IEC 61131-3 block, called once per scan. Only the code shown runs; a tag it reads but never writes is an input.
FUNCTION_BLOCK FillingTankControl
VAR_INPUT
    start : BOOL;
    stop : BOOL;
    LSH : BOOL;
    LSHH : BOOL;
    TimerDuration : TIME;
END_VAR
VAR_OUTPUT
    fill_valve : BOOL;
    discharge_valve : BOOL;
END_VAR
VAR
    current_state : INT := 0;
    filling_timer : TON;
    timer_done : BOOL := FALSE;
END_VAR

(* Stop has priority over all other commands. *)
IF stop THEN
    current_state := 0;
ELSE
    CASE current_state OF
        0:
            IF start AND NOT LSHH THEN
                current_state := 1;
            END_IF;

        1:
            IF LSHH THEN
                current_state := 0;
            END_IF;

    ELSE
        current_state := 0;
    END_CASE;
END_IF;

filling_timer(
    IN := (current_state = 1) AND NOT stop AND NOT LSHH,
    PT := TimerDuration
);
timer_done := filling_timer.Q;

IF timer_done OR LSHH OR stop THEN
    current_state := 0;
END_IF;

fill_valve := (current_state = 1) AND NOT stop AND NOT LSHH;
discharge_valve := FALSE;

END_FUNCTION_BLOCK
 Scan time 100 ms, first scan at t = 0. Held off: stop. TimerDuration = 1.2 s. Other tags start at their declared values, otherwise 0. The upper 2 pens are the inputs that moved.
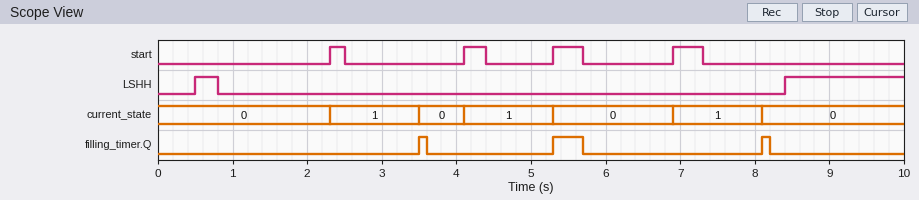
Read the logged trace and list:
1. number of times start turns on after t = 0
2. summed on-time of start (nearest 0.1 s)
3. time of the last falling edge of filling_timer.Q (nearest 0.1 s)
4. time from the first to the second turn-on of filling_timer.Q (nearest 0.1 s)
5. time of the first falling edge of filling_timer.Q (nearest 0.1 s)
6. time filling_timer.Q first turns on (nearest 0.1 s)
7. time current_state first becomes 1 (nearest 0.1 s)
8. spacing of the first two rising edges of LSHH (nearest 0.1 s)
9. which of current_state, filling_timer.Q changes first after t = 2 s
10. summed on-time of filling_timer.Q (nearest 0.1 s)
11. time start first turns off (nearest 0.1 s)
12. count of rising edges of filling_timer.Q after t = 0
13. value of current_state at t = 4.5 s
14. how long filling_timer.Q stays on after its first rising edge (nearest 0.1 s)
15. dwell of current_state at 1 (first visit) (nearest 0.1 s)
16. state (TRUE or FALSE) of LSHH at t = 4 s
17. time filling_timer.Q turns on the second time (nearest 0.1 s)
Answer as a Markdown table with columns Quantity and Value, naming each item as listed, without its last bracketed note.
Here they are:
| Quantity | Value |
|---|---|
| number of times start turns on after t = 0 | 4 |
| summed on-time of start | 1.3 s |
| time of the last falling edge of filling_timer.Q | 8.2 s |
| time from the first to the second turn-on of filling_timer.Q | 1.8 s |
| time of the first falling edge of filling_timer.Q | 3.6 s |
| time filling_timer.Q first turns on | 3.5 s |
| time current_state first becomes 1 | 2.3 s |
| spacing of the first two rising edges of LSHH | 7.9 s |
| which of current_state, filling_timer.Q changes first after t = 2 s | current_state |
| summed on-time of filling_timer.Q | 0.6 s |
| time start first turns off | 2.5 s |
| count of rising edges of filling_timer.Q after t = 0 | 3 |
| value of current_state at t = 4.5 s | 1 |
| how long filling_timer.Q stays on after its first rising edge | 0.1 s |
| dwell of current_state at 1 (first visit) | 1.2 s |
| state (TRUE or FALSE) of LSHH at t = 4 s | FALSE |
| time filling_timer.Q turns on the second time | 5.3 s |
